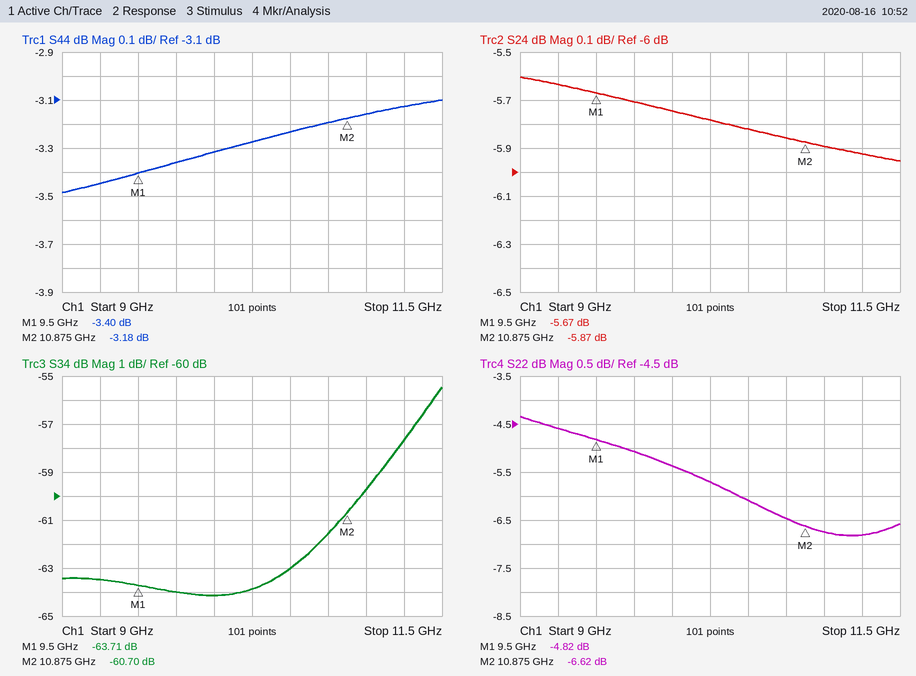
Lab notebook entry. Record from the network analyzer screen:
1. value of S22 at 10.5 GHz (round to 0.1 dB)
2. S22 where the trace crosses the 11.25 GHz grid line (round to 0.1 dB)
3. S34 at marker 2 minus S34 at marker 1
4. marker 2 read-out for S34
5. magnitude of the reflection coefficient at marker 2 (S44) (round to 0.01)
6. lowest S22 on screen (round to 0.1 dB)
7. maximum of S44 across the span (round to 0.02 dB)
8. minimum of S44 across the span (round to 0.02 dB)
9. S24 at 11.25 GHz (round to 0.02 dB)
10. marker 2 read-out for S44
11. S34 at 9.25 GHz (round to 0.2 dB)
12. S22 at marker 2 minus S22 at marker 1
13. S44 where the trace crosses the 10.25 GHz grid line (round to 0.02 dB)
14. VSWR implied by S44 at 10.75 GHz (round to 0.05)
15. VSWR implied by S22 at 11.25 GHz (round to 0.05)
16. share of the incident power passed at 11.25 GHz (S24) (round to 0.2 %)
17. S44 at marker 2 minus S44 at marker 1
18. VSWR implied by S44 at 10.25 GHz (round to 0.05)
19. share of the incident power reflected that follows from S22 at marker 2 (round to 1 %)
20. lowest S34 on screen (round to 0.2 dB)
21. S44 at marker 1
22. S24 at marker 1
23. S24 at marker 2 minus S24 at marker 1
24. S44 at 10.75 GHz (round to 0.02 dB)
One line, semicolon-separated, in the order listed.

-6.1 dB; -6.8 dB; 3.01 dB; -60.70 dB; 0.69; -6.8 dB; -3.10 dB; -3.48 dB; -5.92 dB; -3.18 dB; -63.4 dB; -1.80 dB; -3.28 dB; 5.50; 2.70; 25.6 %; 0.22 dB; 5.35; 22 %; -64.2 dB; -3.40 dB; -5.67 dB; -0.20 dB; -3.20 dB
